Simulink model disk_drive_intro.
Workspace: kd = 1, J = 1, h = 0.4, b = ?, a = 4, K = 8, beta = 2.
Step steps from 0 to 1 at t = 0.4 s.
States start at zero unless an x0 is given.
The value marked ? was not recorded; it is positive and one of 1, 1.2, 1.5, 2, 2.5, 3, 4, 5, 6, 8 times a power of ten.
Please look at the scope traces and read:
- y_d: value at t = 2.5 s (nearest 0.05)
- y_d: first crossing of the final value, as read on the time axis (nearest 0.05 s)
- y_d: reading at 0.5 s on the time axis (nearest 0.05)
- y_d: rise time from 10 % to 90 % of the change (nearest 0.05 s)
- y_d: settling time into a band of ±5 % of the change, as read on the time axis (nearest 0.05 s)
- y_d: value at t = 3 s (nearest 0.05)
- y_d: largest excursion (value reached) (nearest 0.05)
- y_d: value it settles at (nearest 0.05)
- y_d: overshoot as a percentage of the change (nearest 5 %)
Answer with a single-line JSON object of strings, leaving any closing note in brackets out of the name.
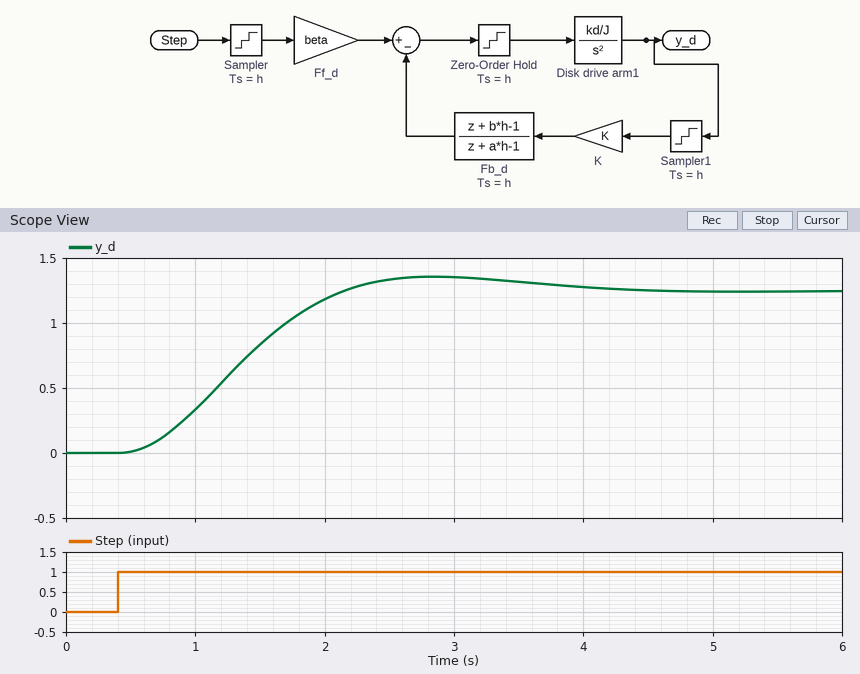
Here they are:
{"y_d: value at t = 2.5 s": "1.35", "y_d: first crossing of the final value, as read on the time axis": "2.15 s", "y_d: reading at 0.5 s on the time axis": "0.00", "y_d: rise time from 10 % to 90 % of the change": "1.15 s", "y_d: settling time into a band of ±5 % of the change, as read on the time axis": "3.55 s", "y_d: value at t = 3 s": "1.35", "y_d: largest excursion (value reached)": "1.35", "y_d: value it settles at": "1.25", "y_d: overshoot as a percentage of the change": "10 %"}
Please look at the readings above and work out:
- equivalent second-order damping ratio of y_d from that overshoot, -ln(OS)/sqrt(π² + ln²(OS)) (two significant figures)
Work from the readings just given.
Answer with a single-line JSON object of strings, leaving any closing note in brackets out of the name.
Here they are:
{"equivalent second-order damping ratio of y_d from that overshoot, -ln(OS)/sqrt(π² + ln²(OS))": "0.59"}
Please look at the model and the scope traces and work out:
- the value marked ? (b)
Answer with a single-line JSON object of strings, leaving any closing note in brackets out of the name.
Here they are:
{"the value marked ?": "0.8"}
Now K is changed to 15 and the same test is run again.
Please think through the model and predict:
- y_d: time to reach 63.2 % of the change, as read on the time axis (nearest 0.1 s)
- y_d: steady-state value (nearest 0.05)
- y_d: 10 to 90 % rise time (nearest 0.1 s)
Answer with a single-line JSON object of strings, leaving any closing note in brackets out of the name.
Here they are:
{"y_d: time to reach 63.2 % of the change, as read on the time axis": "1.2 s", "y_d: steady-state value": "0.65", "y_d: 10 to 90 % rise time": "1.6 s"}
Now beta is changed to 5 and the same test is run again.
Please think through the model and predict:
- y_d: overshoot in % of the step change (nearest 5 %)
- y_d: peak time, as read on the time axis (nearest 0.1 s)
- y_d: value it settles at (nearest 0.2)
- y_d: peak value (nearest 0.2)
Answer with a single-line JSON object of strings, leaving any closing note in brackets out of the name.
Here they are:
{"y_d: overshoot in % of the step change": "10 %", "y_d: peak time, as read on the time axis": "2.8 s", "y_d: value it settles at": "3.2", "y_d: peak value": "3.4"}
